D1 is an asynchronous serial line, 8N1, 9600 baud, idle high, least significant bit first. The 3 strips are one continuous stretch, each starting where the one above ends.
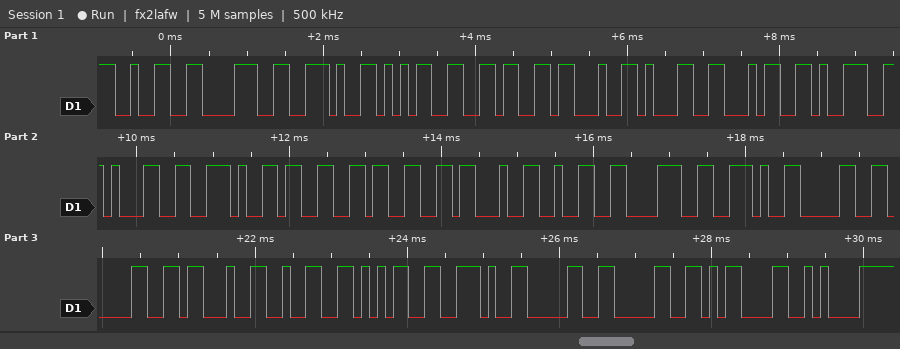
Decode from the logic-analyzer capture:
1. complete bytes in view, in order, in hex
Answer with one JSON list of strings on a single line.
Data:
["32 38 2E 35 36 23 31 34 39 31 2E 33 33 23 32 38 2E 30 30 23 32 35 2E 30 30 0D 0A"]
